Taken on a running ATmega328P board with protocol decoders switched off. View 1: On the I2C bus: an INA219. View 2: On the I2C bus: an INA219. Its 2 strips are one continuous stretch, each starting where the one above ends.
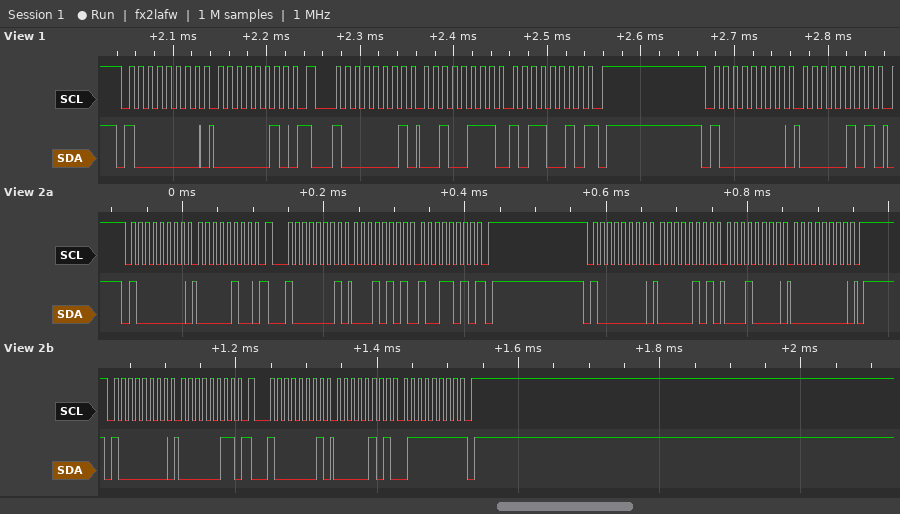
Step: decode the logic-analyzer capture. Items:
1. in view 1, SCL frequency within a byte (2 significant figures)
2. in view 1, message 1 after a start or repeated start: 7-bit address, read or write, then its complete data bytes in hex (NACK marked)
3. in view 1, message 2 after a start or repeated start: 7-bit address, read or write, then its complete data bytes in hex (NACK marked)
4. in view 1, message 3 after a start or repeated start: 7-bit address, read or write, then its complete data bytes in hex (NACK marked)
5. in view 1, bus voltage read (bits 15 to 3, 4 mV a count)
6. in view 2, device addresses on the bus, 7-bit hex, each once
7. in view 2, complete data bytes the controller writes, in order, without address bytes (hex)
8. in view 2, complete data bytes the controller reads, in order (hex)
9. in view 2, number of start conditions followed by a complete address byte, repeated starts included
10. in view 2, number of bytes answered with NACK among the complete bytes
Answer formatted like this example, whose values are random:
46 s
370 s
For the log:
100 kHz
0x40 write: 02
0x40 read: 27 B2 NACK
0x40 write: 05
5.080 V
0x40
04 05 10 00 03
15 9A 05 7F
5
2
